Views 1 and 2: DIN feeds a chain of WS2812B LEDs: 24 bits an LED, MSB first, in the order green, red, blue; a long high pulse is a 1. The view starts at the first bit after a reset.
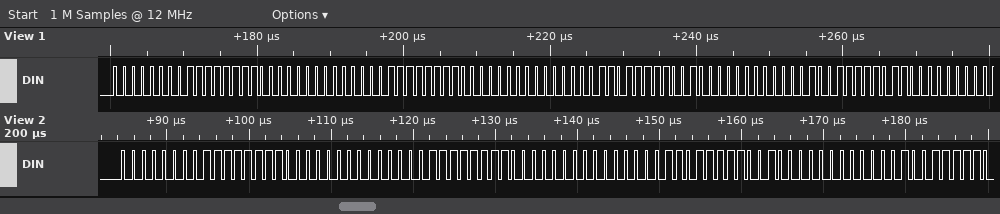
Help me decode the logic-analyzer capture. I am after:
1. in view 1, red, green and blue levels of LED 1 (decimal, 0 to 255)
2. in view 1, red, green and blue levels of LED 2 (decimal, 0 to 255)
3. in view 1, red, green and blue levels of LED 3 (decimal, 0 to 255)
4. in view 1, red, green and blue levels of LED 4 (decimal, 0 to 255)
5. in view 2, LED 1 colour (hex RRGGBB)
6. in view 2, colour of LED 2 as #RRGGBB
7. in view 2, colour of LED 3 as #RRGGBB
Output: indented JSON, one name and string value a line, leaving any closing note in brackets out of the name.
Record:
{
  "in view 1, red, green and blue levels of LED 1": "255, 0, 0",
  "in view 1, red, green and blue levels of LED 2": "252, 3, 0",
  "in view 1, red, green and blue levels of LED 3": "249, 6, 0",
  "in view 1, red, green and blue levels of LED 4": "246, 9, 0",
  "in view 2, LED 1 colour": "#FF0000",
  "in view 2, colour of LED 2 as #RRGGBB": "#FC0300",
  "in view 2, colour of LED 3 as #RRGGBB": "#F90600"
}
